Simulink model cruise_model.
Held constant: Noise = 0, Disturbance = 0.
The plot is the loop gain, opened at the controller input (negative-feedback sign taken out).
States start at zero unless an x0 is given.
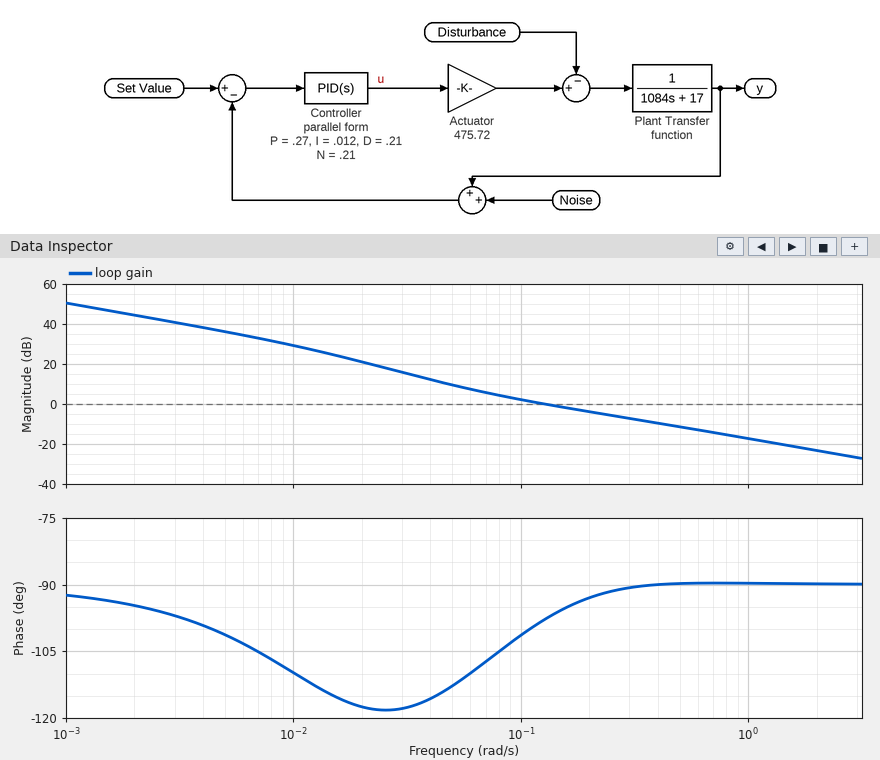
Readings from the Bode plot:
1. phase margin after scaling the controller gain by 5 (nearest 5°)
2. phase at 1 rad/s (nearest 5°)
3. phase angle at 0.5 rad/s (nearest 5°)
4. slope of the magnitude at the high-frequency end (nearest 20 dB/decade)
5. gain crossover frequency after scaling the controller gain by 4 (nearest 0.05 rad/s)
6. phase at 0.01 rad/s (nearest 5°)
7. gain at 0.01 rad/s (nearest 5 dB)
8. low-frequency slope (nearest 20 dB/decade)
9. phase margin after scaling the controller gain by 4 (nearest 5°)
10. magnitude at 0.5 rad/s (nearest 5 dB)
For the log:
90°
-90°
-90°
-20 dB/decade
0.55 rad/s
-110°
30 dB
-20 dB/decade
90°
-10 dB
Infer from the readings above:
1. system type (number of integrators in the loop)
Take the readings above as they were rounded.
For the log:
1
